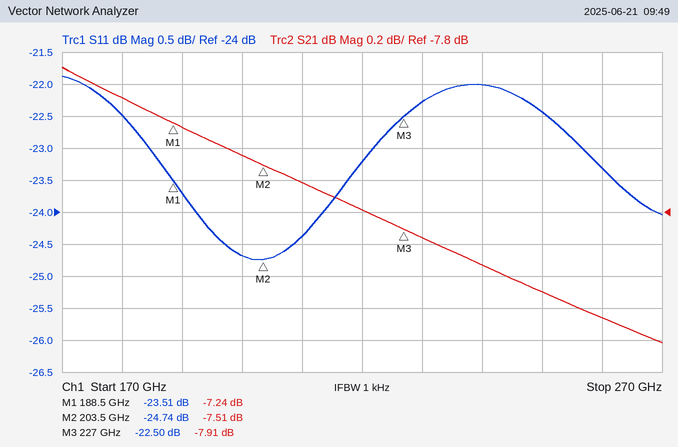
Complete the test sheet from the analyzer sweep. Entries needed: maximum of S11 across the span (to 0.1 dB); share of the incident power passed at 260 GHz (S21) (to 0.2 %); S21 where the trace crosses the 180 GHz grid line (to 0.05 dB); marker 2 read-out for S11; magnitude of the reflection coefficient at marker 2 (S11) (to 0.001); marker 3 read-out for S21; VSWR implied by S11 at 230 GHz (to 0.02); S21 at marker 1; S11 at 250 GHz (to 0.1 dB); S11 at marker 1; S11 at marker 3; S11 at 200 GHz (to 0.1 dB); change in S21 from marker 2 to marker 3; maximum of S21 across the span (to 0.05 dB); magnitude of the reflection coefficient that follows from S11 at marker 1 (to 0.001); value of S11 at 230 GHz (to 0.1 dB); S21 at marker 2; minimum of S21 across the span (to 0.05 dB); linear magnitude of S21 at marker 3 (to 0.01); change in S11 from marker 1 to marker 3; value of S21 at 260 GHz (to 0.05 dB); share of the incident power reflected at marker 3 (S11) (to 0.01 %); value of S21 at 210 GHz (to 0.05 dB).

-21.9 dB
14.2 %
-7.10 dB
-24.74 dB
0.058
-7.91 dB
1.16
-7.24 dB
-22.4 dB
-23.51 dB
-22.50 dB
-24.7 dB
-0.40 dB
-6.90 dB
0.067
-22.3 dB
-7.51 dB
-8.60 dB
0.40
1.01 dB
-8.45 dB
0.56 %
-7.60 dB
